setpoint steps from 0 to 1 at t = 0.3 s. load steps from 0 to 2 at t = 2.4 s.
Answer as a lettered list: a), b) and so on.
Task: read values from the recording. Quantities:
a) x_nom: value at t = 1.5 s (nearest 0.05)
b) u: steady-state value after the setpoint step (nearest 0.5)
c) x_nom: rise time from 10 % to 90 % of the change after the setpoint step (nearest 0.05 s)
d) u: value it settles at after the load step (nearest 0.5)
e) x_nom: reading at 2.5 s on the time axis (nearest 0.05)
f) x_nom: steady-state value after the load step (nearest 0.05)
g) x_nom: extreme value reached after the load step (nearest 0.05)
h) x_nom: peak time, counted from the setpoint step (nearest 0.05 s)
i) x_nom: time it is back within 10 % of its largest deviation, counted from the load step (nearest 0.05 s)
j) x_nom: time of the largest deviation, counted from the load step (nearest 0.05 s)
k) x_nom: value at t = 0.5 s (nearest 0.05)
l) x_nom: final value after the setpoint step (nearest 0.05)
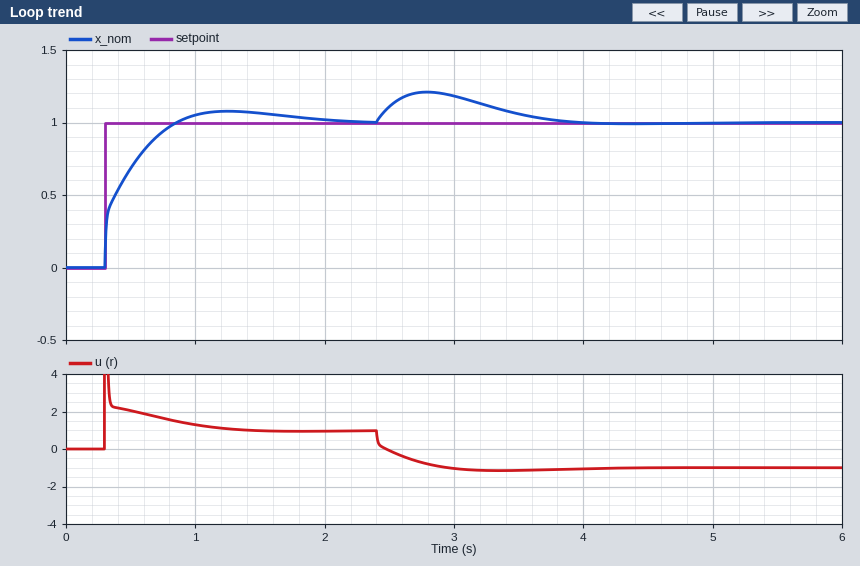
a) 1.05
b) 1.0
c) 0.40 s
d) -1.0
e) 1.10
f) 1.00
g) 1.20
h) 0.95 s
i) 1.35 s
j) 0.40 s
k) 0.70
l) 1.00
